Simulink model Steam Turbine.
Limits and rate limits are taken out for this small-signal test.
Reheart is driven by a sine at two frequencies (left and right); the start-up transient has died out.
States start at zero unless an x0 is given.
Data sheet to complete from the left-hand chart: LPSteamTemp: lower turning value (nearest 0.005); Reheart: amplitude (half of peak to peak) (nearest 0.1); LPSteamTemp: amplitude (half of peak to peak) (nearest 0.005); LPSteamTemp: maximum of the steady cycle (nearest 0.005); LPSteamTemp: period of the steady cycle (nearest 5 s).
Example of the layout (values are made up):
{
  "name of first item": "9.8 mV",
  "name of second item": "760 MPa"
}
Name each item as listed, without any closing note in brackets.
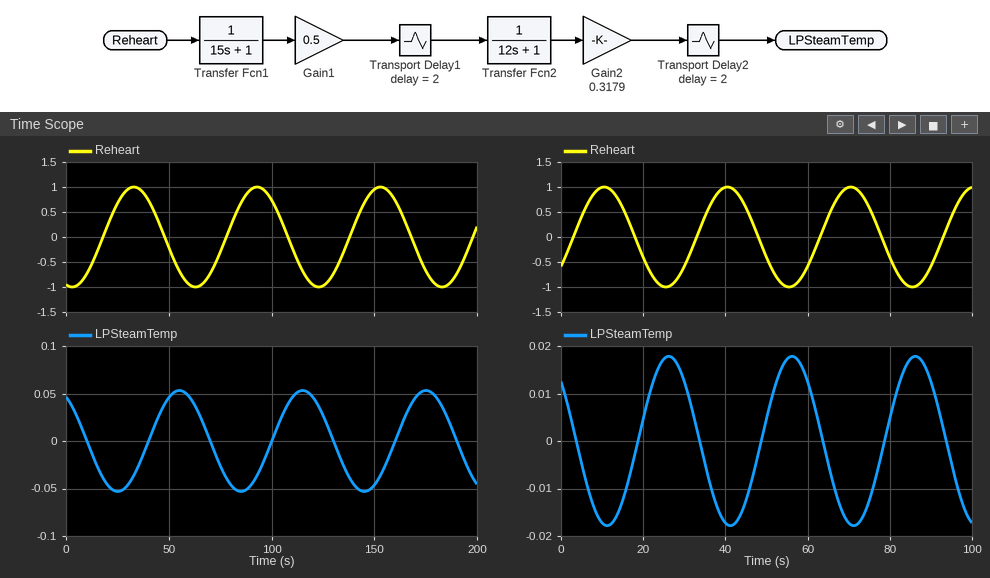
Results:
{
  "LPSteamTemp: lower turning value": "-0.055",
  "Reheart: amplitude (half of peak to peak)": "1.0",
  "LPSteamTemp: amplitude (half of peak to peak)": "0.055",
  "LPSteamTemp: maximum of the steady cycle": "0.055",
  "LPSteamTemp: period of the steady cycle": "60 s"
}
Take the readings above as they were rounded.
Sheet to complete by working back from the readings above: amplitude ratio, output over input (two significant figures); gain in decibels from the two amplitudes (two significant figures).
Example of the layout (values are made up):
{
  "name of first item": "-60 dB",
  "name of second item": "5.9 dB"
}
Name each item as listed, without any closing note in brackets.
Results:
{
  "amplitude ratio, output over input": "0.055",
  "gain in decibels from the two amplitudes": "-25 dB"
}
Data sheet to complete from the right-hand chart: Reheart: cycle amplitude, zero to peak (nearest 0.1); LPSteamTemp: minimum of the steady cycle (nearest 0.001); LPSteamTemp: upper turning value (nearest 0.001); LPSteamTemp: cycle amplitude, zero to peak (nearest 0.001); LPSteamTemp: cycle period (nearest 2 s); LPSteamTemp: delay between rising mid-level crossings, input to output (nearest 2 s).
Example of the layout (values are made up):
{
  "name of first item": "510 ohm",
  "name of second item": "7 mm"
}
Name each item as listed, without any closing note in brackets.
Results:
{
  "Reheart: cycle amplitude, zero to peak": "1.0",
  "LPSteamTemp: minimum of the steady cycle": "-0.018",
  "LPSteamTemp: upper turning value": "0.018",
  "LPSteamTemp: cycle amplitude, zero to peak": "0.018",
  "LPSteamTemp: cycle period": "30 s",
  "LPSteamTemp: delay between rising mid-level crossings, input to output": "16 s"
}
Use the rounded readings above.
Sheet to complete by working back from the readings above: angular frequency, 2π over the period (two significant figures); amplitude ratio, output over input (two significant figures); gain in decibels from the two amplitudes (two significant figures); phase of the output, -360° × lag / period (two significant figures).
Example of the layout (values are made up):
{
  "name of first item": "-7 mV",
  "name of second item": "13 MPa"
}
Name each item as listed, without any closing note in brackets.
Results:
{
  "angular frequency, 2π over the period": "0.21 rad/s",
  "amplitude ratio, output over input": "0.018",
  "gain in decibels from the two amplitudes": "-35 dB",
  "phase of the output, -360° × lag / period": "-190°"
}
